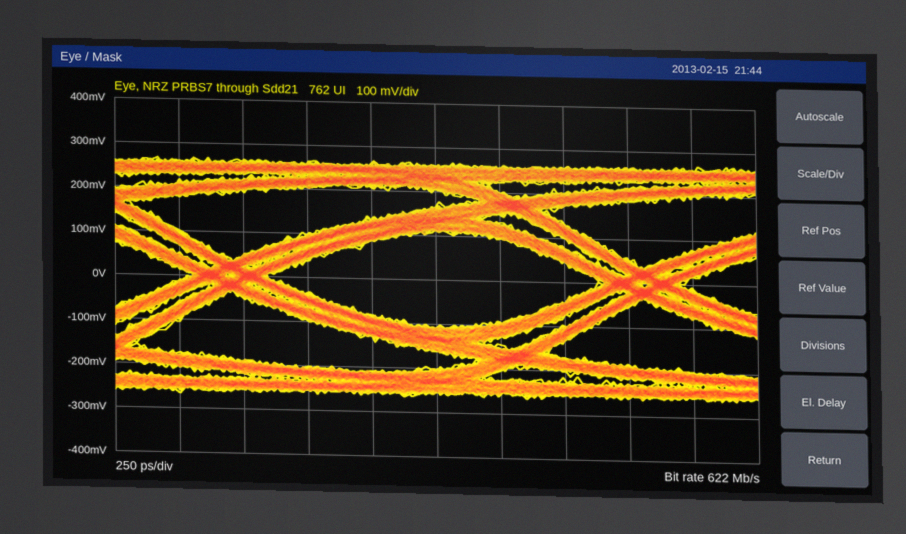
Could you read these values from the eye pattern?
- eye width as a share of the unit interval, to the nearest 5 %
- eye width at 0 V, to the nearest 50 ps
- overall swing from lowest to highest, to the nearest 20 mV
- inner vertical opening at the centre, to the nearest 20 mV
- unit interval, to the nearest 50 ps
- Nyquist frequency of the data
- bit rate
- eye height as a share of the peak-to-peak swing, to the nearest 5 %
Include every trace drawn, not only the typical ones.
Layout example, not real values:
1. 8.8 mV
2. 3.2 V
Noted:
1. 80 %
2. 1.30 ns
3. 540 mV
4. 220 mV
5. 1.60 ns
6. 311 MHz
7. 622 Mb/s
8. 40 %
